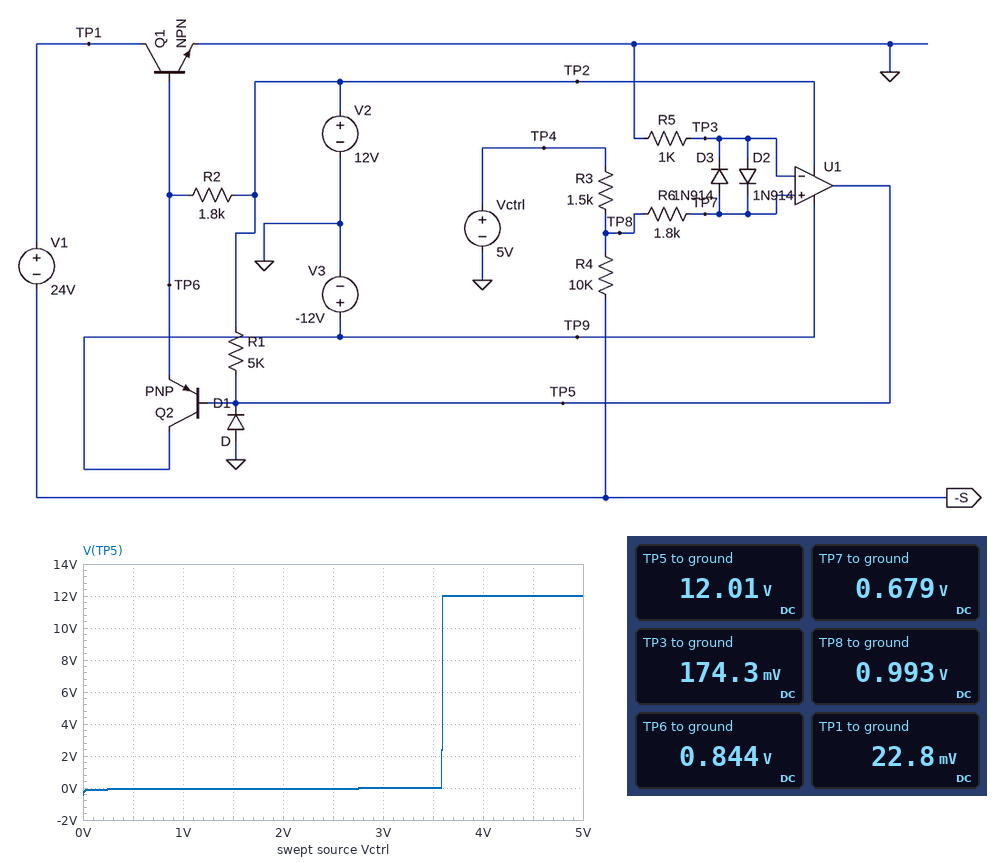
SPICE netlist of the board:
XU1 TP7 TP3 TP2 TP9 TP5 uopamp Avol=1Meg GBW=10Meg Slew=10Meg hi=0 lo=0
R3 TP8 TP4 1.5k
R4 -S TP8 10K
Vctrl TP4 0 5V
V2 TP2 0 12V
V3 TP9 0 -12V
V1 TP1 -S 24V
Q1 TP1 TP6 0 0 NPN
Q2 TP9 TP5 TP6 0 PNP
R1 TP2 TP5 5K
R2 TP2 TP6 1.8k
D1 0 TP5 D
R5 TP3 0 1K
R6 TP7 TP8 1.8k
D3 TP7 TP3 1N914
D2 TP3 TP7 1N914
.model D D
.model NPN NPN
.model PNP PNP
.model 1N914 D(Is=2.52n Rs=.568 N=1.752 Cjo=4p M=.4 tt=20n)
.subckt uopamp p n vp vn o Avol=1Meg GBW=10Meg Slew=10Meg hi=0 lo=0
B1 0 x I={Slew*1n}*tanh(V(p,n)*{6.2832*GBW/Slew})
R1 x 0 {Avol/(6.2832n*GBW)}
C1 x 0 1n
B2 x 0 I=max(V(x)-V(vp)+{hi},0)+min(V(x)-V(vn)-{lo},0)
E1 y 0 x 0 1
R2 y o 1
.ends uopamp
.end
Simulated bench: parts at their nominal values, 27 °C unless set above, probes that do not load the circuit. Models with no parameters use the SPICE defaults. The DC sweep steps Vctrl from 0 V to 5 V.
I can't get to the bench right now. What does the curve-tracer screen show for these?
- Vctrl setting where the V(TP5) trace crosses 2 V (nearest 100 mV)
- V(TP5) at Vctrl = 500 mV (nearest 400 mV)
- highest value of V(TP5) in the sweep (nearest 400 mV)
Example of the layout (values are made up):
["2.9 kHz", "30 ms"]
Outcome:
["3.6 V", "0 V", "12.0 V"]
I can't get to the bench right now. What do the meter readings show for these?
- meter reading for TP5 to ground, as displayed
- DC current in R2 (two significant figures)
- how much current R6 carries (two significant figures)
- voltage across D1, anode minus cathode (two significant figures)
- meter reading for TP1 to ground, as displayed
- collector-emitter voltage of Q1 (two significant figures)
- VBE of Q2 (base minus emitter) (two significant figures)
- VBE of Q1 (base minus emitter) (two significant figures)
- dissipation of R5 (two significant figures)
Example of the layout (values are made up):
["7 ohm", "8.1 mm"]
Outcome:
["12.01 V", "6.2 mA", "170 µA", "-12 V", "22.8 mV", "23 mV", "11 V", "840 mV", "30 µW"]
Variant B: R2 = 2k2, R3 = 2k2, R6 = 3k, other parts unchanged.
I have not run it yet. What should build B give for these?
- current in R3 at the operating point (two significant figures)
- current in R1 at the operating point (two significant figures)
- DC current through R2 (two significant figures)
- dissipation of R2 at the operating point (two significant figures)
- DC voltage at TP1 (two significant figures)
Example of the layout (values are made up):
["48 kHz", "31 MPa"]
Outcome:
["2.3 mA", "2.4 mA", "5.1 mA", "57 mW", "1.3 V"]
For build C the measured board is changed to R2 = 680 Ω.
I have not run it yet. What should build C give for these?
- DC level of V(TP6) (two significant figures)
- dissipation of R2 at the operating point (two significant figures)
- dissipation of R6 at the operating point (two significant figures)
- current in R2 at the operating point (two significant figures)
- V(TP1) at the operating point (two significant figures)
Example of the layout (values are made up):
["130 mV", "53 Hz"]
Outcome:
["870 mV", "180 mW", "55 µW", "16 mA", "20 mV"]
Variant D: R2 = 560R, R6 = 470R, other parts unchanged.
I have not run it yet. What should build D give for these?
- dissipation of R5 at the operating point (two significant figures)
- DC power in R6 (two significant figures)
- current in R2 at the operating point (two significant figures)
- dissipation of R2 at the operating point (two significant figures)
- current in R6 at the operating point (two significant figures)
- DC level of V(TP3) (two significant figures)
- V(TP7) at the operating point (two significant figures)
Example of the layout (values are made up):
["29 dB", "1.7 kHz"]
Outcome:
["63 µW", "30 µW", "20 mA", "220 mW", "250 µA", "250 mV", "770 mV"]
